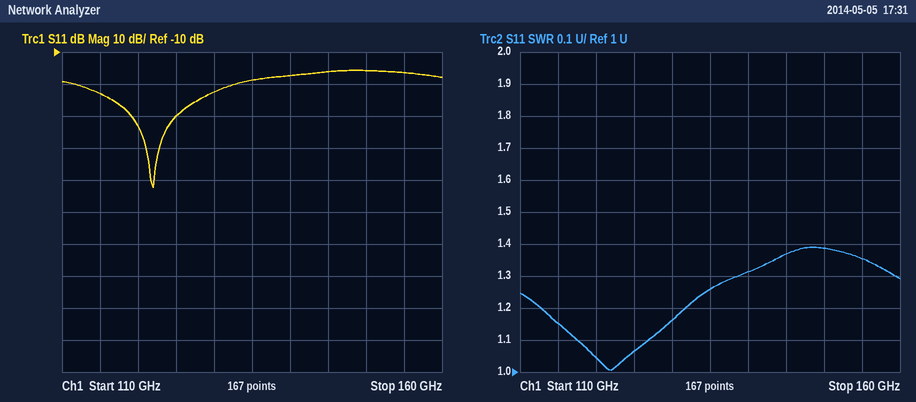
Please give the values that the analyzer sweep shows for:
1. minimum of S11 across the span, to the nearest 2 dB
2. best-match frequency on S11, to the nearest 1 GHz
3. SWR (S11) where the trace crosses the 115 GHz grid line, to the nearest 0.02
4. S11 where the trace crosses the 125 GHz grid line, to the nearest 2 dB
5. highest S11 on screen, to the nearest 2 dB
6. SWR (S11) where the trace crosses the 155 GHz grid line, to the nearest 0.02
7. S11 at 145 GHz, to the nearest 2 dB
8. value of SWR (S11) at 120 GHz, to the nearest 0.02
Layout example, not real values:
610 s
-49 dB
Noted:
-52 dB
122 GHz
1.16
-30 dB
-16 dB
1.36
-16 dB
1.04
